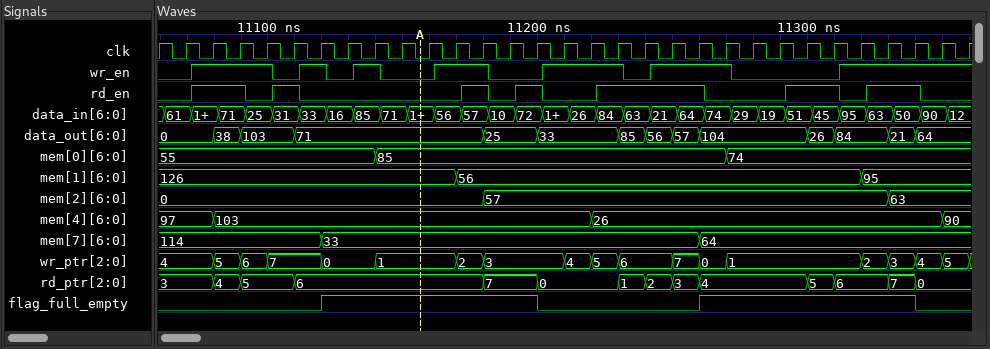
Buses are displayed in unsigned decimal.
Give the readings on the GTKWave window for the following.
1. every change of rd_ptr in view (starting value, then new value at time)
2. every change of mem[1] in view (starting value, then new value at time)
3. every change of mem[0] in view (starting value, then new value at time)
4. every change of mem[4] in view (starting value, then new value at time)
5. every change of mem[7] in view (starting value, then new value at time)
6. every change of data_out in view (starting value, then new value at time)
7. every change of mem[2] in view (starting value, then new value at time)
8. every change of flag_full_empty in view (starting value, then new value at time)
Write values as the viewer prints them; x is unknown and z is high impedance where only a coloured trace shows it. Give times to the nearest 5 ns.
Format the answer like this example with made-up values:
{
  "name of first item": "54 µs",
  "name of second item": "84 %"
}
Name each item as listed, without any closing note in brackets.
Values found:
{
  "every change of rd_ptr in view": "3, 4 at 11080 ns, 5 at 11090 ns, 6 at 11110 ns, 7 at 11180 ns, 0 at 11200 ns, 1 at 11230 ns, 2 at 11240 ns, 3 at 11250 ns, 4 at 11260 ns, 5 at 11300 ns, 6 at 11310 ns, 7 at 11330 ns, 0 at 11340 ns",
  "every change of mem[1] in view": "126, 56 at 11170 ns, 95 at 11320 ns",
  "every change of mem[0] in view": "55, 85 at 11140 ns, 74 at 11270 ns",
  "every change of mem[4] in view": "97, 103 at 11080 ns, 26 at 11220 ns, 90 at 11350 ns",
  "every change of mem[7] in view": "114, 33 at 11120 ns, 64 at 11260 ns",
  "every change of data_out in view": "0, 38 at 11080 ns, 103 at 11090 ns, 71 at 11110 ns, 25 at 11180 ns, 33 at 11200 ns, 85 at 11230 ns, 56 at 11240 ns, 57 at 11250 ns, 104 at 11260 ns, 26 at 11300 ns, 84 at 11310 ns, 21 at 11330 ns, 64 at 11340 ns",
  "every change of mem[2] in view": "0, 57 at 11180 ns, 63 at 11330 ns",
  "every change of flag_full_empty in view": "0, 1 at 11120 ns, 0 at 11200 ns, 1 at 11260 ns, 0 at 11340 ns"
}
